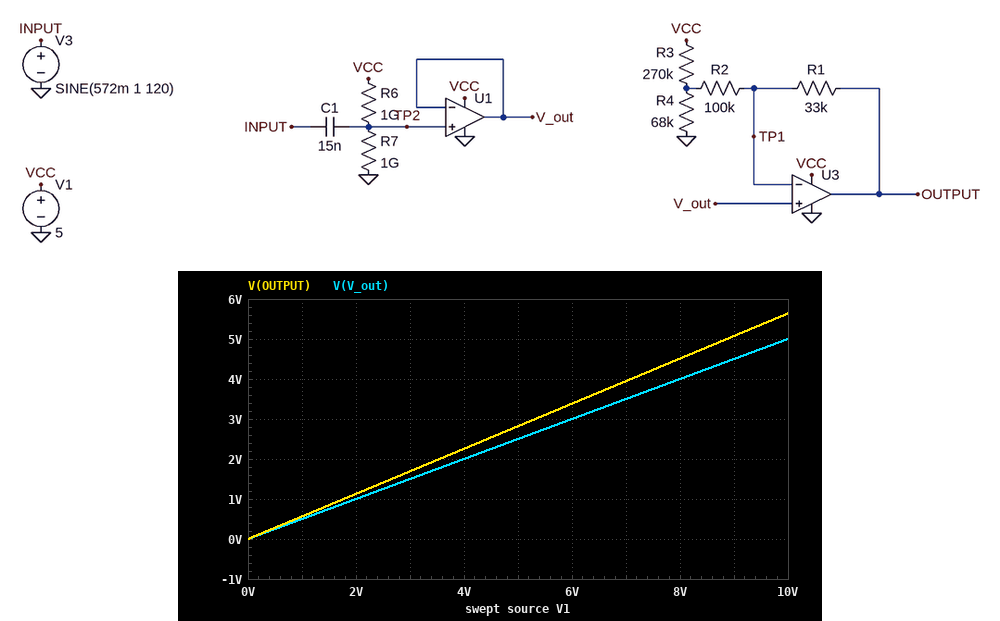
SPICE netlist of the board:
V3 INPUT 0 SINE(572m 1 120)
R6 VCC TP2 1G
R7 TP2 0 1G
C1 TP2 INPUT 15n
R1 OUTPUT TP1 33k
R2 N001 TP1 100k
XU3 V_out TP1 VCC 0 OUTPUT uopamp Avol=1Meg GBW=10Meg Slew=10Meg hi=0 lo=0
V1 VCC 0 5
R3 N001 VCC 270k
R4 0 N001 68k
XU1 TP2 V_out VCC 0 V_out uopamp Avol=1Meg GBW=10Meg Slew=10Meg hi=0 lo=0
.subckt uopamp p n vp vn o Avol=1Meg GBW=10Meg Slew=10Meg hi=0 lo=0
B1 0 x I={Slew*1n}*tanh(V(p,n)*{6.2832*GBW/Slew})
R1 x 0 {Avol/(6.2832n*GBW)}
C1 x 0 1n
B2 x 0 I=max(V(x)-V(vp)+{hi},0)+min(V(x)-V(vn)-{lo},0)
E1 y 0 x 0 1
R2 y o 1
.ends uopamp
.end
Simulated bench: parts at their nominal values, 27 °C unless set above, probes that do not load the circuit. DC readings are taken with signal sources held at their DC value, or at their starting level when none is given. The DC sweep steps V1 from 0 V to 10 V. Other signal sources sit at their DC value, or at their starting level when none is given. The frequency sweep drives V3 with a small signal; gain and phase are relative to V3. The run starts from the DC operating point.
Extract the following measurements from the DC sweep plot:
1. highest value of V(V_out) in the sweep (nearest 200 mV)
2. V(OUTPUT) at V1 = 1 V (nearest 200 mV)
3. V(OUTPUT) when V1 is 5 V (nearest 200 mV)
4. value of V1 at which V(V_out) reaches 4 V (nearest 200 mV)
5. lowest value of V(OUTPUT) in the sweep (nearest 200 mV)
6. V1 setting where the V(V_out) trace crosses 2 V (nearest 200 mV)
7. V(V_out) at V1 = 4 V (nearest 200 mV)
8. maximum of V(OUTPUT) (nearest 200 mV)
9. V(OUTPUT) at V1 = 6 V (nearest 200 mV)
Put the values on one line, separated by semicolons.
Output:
5.0 V; 600 mV; 2.8 V; 8.0 V; 0 V; 4.0 V; 2.0 V; 5.6 V; 3.4 V
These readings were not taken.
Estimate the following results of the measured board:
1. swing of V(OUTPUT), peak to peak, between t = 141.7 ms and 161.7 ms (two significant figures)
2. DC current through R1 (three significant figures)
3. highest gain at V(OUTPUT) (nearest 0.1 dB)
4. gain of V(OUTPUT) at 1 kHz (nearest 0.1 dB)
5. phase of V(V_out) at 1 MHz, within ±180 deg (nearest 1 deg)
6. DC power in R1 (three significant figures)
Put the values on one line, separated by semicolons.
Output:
2.4 V; 9.68 µA; 1.7 dB; 1.7 dB; -6 deg; 3.09 µW
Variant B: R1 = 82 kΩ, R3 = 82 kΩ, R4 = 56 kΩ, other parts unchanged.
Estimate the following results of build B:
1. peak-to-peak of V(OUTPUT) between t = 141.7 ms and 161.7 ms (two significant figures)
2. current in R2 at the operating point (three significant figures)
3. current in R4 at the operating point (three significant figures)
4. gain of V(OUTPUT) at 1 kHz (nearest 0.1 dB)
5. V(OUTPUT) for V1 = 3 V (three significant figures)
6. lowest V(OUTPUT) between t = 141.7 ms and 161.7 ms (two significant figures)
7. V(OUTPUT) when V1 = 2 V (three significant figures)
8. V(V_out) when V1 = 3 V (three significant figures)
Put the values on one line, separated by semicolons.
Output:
3.2 V; 3.53 µA; 38.3 µA; 4.2 dB; 1.67 V; 1.2 V; 1.12 V; 1.50 V
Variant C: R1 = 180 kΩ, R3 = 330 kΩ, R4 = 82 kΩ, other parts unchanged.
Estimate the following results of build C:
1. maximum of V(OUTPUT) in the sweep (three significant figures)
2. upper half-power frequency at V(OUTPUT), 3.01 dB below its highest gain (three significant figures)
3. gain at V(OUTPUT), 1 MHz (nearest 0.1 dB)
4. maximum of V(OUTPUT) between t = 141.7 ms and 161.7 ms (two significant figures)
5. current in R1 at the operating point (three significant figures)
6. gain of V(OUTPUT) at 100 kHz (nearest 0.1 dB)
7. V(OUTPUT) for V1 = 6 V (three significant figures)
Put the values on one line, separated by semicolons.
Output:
8.27 V; 4.06 MHz; 6.2 dB; 5.0 V; 9.08 µA; 6.4 dB; 4.96 V
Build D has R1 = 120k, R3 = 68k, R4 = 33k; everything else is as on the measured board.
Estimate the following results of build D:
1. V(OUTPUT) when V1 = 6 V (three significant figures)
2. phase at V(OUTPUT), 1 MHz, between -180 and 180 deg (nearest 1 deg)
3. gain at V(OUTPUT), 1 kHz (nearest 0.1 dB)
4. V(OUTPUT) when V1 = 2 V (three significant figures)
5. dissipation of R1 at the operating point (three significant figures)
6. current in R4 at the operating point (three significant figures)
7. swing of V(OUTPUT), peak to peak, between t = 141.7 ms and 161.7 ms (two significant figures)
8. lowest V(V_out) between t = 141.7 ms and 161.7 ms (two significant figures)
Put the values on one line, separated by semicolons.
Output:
4.02 V; -17 deg; 5.9 dB; 1.34 V; 6.03 µW; 54.3 µA; 3.6 V; 1.5 V
